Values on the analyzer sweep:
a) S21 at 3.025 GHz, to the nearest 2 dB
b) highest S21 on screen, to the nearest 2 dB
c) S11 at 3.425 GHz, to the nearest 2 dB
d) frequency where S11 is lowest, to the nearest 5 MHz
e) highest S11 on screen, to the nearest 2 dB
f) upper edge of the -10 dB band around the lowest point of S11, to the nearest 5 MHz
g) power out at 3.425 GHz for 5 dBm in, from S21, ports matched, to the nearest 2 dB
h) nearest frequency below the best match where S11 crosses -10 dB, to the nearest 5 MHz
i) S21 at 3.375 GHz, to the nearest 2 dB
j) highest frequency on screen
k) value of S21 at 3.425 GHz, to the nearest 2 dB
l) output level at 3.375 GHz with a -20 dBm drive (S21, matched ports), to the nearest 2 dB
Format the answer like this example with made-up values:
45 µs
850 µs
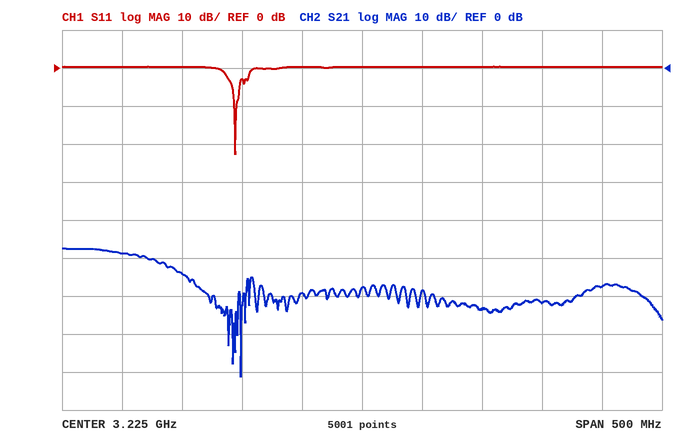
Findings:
-48 dB
-48 dB
0 dB
3.120 GHz
0 dB
3.120 GHz
-52 dBm
3.120 GHz
-62 dB
3.475 GHz
-58 dB
-82 dBm
